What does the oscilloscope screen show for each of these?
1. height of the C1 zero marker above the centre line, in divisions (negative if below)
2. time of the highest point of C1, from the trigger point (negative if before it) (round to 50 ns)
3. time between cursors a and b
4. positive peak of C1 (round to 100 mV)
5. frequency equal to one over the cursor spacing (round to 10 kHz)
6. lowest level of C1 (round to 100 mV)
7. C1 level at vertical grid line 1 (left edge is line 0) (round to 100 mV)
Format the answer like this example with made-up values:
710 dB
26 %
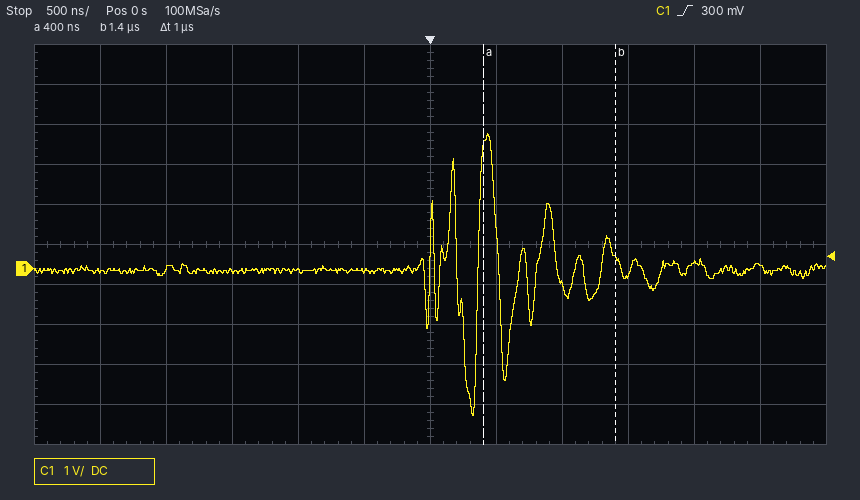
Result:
-0.6 div
+450 ns
1 µs
3.4 V
1.00 MHz
-3.7 V
-100 mV
